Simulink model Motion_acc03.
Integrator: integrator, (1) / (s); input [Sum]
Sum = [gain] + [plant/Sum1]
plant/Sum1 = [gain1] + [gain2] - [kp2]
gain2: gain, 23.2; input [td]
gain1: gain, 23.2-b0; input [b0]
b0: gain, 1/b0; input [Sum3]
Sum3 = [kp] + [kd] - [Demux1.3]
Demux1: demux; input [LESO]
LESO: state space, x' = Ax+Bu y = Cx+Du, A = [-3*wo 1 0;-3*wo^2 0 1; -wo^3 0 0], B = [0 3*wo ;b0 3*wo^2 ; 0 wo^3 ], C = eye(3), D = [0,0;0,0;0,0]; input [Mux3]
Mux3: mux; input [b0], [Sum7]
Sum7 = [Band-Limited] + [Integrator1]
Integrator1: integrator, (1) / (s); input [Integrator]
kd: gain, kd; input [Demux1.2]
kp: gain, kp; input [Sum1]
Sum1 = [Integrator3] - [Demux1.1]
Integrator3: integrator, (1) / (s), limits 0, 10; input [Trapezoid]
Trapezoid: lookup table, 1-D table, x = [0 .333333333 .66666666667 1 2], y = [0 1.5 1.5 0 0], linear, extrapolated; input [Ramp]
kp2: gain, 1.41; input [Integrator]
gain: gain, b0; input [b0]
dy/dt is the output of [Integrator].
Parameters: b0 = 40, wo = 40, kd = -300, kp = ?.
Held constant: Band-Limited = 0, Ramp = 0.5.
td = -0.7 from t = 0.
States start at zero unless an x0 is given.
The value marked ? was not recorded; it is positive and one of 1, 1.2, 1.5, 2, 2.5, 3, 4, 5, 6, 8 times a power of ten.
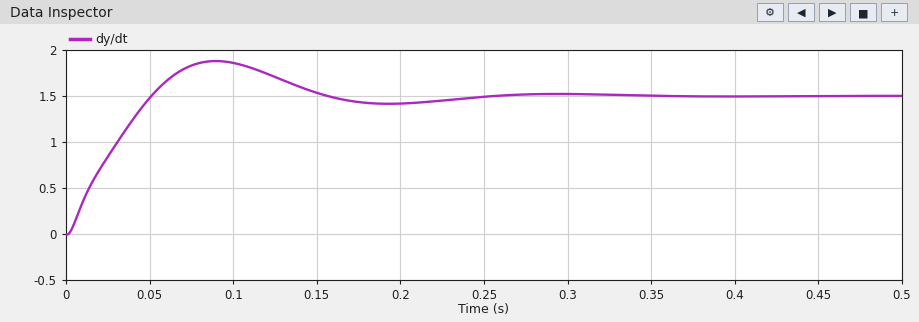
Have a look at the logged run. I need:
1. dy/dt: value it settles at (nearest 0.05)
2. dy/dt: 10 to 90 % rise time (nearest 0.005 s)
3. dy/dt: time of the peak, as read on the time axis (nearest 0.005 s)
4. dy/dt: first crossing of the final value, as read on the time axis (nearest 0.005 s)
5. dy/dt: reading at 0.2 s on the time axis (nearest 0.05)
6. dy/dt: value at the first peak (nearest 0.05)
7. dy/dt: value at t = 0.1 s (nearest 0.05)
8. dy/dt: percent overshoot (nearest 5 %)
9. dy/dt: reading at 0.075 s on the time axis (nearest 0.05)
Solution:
1.50
0.040 s
0.090 s
0.050 s
1.40
1.90
1.85
25 %
1.85
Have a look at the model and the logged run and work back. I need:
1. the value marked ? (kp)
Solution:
30000
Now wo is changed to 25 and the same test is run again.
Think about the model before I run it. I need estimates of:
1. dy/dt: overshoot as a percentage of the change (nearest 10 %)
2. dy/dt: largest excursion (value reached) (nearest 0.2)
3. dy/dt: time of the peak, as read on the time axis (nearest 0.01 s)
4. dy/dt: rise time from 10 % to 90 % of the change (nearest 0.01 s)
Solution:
20 %
1.8
0.14 s
0.06 s
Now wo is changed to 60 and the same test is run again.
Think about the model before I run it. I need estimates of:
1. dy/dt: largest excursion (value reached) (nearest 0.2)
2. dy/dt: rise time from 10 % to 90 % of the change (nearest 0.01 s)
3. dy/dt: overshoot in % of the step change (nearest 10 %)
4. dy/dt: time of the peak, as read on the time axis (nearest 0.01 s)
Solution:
2.0
0.03 s
30 %
0.07 s
